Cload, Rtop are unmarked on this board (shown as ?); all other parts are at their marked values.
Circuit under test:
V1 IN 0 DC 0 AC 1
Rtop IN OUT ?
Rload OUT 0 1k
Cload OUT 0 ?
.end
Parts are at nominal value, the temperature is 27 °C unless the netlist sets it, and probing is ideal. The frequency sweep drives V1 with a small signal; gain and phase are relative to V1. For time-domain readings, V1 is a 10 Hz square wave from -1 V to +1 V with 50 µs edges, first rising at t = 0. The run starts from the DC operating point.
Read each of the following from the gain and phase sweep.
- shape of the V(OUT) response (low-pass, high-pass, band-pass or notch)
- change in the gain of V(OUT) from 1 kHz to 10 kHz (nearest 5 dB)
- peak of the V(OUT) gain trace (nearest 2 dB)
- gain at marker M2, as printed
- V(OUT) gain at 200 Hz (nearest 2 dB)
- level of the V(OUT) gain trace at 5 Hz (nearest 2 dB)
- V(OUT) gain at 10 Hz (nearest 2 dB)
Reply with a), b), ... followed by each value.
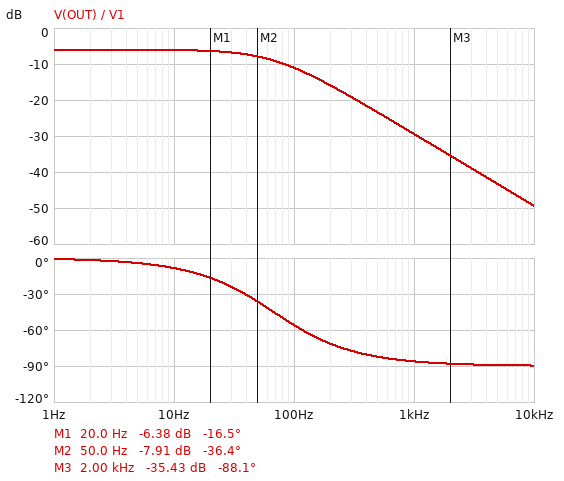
a) low-pass
b) -20 dB
c) -6 dB
d) -7.91 dB
e) -16 dB
f) -6 dB
g) -6 dB
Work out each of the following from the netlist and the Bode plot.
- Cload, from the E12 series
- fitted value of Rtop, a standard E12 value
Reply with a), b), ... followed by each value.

a) 4.7 µF
b) 1 kΩ
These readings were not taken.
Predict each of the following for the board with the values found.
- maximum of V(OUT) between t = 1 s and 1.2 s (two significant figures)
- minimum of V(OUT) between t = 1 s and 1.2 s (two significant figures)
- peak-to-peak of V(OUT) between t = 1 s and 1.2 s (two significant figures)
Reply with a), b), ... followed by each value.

a) 500 mV
b) -500 mV
c) 1.0 V
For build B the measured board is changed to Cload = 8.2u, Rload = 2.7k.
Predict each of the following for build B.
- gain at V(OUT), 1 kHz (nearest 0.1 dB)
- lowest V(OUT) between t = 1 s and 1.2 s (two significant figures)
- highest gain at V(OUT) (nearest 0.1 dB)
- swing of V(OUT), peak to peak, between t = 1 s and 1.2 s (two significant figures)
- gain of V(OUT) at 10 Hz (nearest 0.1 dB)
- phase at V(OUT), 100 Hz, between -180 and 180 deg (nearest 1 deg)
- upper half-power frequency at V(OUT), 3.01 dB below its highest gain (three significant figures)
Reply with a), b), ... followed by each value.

a) -34.2 dB
b) -730 mV
c) -2.7 dB
d) 1.5 V
e) -3.3 dB
f) -75 deg
g) 26.6 Hz
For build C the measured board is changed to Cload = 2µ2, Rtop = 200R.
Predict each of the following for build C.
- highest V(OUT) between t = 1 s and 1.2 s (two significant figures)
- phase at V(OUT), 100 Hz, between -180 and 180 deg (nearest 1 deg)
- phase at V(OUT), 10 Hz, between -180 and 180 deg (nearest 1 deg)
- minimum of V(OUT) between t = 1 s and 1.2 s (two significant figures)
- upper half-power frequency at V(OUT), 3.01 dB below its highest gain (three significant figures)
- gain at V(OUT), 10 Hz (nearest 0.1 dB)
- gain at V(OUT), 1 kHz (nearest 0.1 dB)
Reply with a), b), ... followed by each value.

a) 830 mV
b) -13 deg
c) -1 deg
d) -830 mV
e) 434 Hz
f) -1.6 dB
g) -9.6 dB
